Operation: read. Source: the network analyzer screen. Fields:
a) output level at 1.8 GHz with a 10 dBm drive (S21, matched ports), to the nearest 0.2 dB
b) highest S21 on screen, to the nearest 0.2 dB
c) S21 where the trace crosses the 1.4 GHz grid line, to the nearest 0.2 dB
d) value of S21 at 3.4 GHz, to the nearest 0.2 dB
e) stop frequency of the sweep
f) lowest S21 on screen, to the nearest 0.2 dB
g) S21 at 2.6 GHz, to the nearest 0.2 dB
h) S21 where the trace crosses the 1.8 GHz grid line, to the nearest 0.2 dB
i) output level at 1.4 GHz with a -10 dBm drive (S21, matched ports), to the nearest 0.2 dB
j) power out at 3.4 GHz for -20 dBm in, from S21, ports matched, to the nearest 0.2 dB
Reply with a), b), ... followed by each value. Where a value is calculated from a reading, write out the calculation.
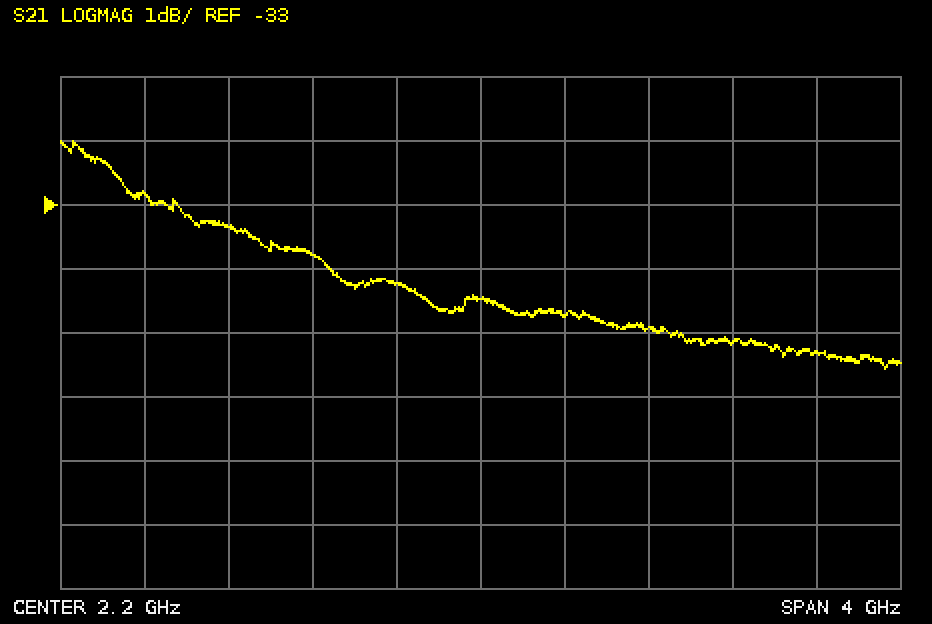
a) 10 dBm + (-34.2 dB) = -24.2 dBm
b) -32.0 dB
c) -33.8 dB
d) -35.2 dB
e) 4.2 GHz
f) -35.6 dB
g) -34.8 dB
h) -34.2 dB
i) -10 dBm + (-33.8 dB) = -43.8 dBm
j) -20 dBm + (-35.2 dB) = -55.2 dBm
